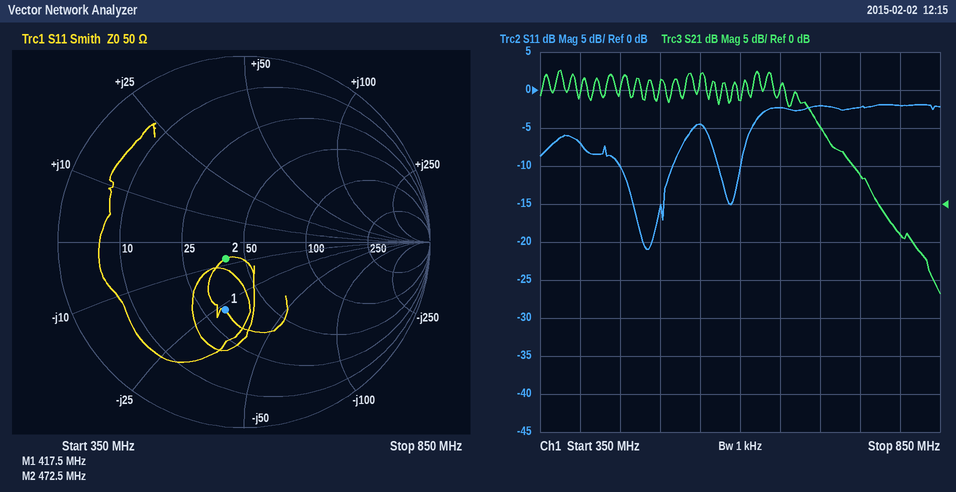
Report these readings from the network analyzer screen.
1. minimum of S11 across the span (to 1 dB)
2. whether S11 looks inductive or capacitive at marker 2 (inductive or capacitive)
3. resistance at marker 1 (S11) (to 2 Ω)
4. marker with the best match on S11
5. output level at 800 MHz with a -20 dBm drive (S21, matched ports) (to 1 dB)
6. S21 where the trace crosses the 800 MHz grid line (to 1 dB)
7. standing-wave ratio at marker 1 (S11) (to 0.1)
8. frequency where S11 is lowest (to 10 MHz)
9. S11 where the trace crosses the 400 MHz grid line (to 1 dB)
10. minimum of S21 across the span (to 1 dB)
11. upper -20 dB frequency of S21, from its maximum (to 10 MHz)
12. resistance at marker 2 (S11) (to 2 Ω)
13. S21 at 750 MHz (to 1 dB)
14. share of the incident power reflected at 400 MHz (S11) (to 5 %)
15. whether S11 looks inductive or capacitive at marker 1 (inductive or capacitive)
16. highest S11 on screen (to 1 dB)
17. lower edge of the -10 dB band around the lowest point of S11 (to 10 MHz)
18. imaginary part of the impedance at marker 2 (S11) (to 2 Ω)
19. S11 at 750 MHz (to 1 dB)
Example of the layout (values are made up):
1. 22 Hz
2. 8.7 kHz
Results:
1. -21 dB
2. capacitive
3. 32 Ω
4. marker 2
5. -24 dBm
6. -4 dB
7. 2.2
8. 480 MHz
9. -7 dB
10. -12 dB
11. 790 MHz
12. 40 Ω
13. 4 dB
14. 20 %
15. capacitive
16. -2 dB
17. 450 MHz
18. -8 Ω
19. -2 dB
